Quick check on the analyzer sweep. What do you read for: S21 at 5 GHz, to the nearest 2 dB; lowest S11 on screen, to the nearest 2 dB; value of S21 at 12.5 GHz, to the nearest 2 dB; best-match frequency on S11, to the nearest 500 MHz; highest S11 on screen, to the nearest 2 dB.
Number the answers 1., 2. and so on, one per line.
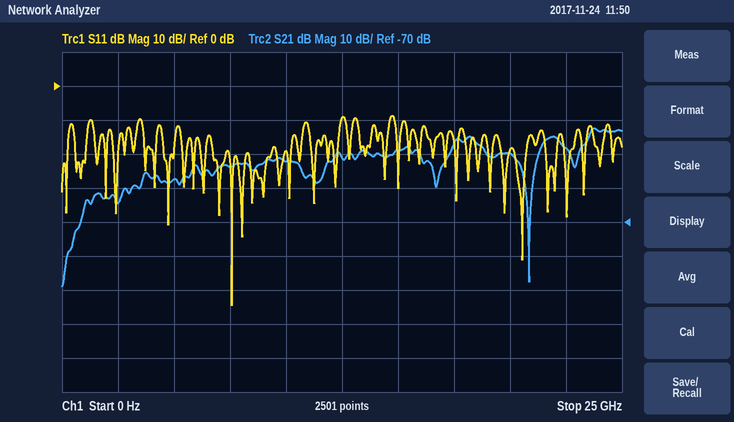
1. -58 dB
2. -64 dB
3. -52 dB
4. 7.5 GHz
5. -8 dB
